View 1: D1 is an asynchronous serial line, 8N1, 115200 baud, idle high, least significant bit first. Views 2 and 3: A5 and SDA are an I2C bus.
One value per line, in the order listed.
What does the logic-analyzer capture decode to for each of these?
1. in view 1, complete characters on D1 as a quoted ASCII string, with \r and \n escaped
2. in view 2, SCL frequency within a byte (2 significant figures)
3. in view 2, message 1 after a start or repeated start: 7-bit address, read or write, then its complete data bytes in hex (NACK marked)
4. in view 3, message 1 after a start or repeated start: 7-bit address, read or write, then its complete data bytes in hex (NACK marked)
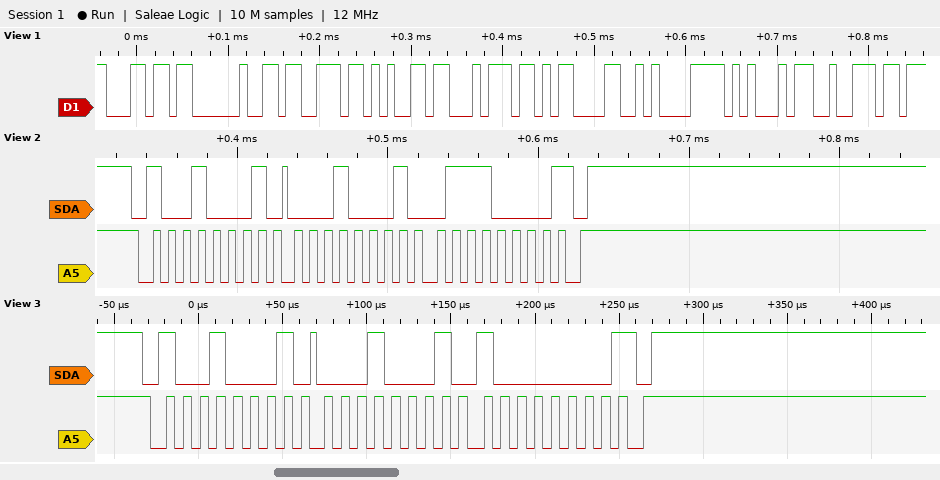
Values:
"l set\r\nEr"
100 kHz
0x48 read: 11 70 NACK
0x48 read: 11 80 NACK
